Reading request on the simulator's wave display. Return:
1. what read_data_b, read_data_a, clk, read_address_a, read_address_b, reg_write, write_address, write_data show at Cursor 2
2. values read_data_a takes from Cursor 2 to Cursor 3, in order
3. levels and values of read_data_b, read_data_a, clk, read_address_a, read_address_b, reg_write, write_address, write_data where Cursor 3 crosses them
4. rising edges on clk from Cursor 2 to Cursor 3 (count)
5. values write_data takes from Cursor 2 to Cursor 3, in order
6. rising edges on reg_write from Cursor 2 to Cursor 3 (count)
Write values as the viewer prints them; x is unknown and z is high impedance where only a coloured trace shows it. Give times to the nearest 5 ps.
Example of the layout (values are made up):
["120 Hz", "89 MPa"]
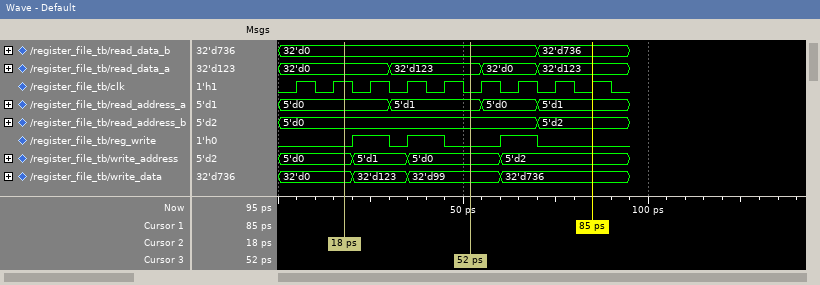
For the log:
["read_data_b=32'd0, read_data_a=32'd0, clk=1, read_address_a=5'd0, read_address_b=5'd0, reg_write=0, write_address=5'd0, write_data=32'd0", "32'd0, 32'd123", "read_data_b=32'd0, read_data_a=32'd123, clk=0, read_address_a=5'd1, read_address_b=5'd0, reg_write=0, write_address=5'd0, write_data=32'd99", "3", "32'd0, 32'd123, 32'd99", "2"]
